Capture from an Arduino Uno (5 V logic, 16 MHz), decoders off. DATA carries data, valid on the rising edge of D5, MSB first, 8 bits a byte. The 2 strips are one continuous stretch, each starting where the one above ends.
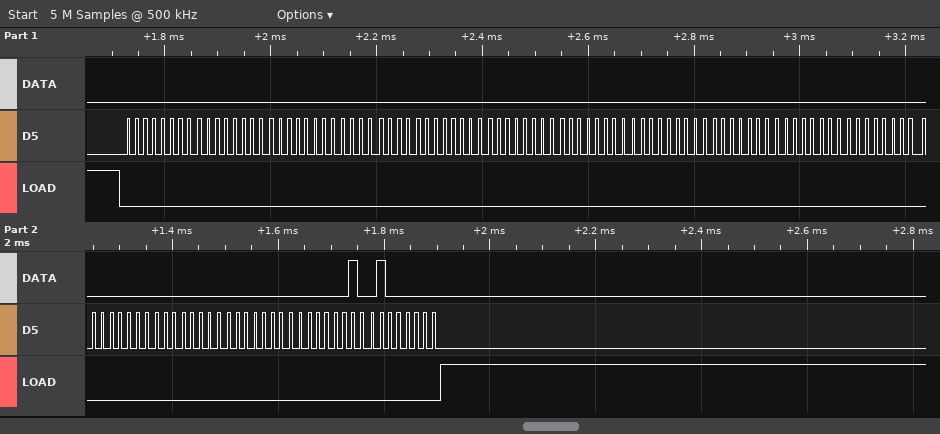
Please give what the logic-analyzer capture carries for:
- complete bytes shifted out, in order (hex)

00 00 00 00 00 00 00 00 00 00 00 00 00 00 02 40
